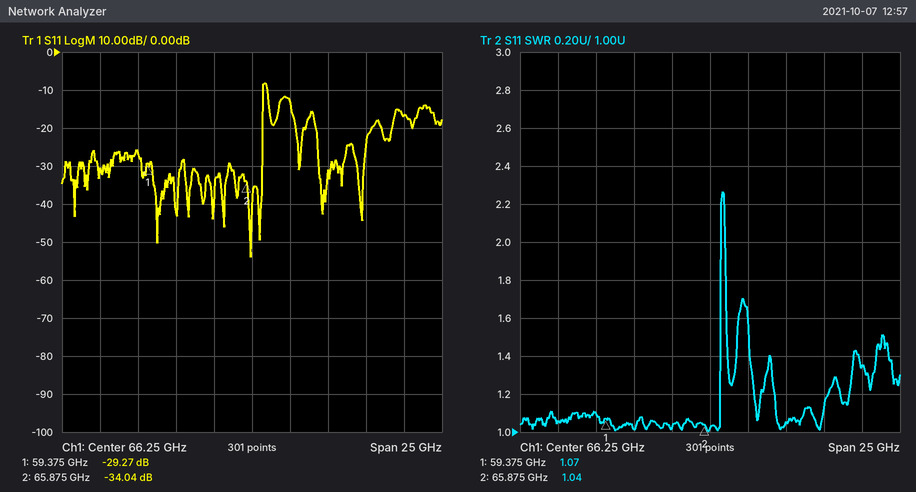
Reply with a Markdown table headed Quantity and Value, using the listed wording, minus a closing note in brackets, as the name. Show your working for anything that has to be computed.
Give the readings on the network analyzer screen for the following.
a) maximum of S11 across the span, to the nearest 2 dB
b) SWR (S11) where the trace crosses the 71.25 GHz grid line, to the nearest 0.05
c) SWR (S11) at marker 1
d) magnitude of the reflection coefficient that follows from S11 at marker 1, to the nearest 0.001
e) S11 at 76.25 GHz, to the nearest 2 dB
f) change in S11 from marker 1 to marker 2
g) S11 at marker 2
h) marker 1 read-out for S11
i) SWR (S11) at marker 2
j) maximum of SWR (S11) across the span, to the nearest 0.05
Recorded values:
| Quantity | Value |
|---|---|
| maximum of S11 across the span, to the nearest 2 dB | -8 dB |
| SWR (S11) where the trace crosses the 71.25 GHz grid line, to the nearest 0.05 | 1.05 |
| SWR (S11) at marker 1 | 1.07 |
| magnitude of the reflection coefficient that follows from S11 at marker 1, to the nearest 0.001 | 10^(-29.27/20) ≈ 0.034 |
| S11 at 76.25 GHz, to the nearest 2 dB | -16 dB |
| change in S11 from marker 1 to marker 2 | -34.04 − (-29.27) = -4.77 dB |
| S11 at marker 2 | -34.04 dB |
| marker 1 read-out for S11 | -29.27 dB |
| SWR (S11) at marker 2 | 1.04 |
| maximum of SWR (S11) across the span, to the nearest 0.05 | 2.25 |
